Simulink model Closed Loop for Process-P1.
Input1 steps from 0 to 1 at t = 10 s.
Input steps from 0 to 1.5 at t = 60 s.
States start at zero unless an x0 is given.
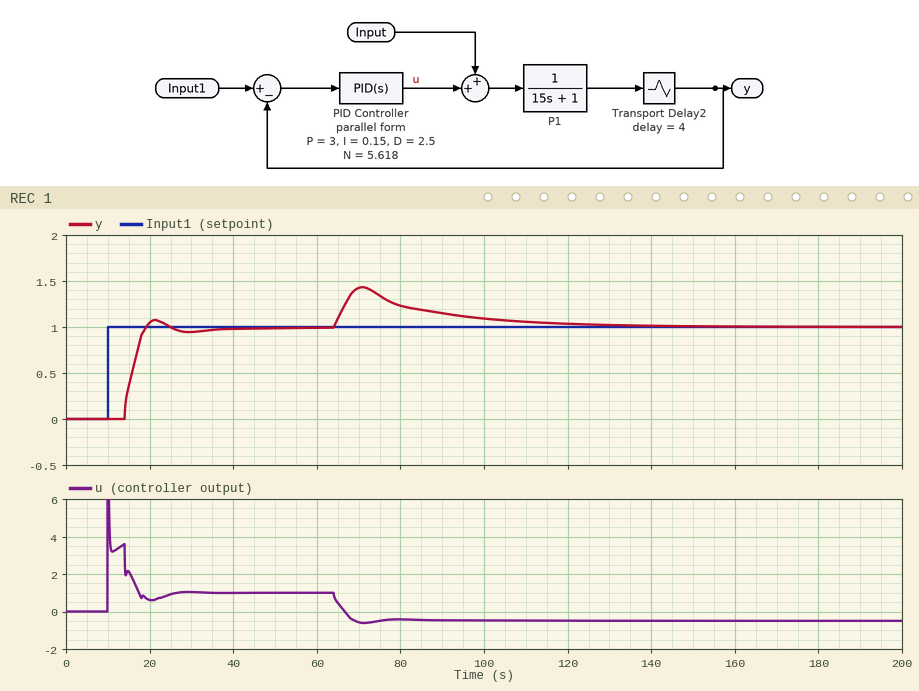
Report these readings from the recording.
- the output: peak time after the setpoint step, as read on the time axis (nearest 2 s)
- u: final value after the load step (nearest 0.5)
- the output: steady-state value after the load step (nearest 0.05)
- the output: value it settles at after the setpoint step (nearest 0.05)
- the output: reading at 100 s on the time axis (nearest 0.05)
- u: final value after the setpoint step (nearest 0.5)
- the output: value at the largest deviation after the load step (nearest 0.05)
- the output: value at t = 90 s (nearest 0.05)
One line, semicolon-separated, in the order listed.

22 s; -0.5; 1.00; 1.00; 1.10; 1.0; 1.45; 1.15
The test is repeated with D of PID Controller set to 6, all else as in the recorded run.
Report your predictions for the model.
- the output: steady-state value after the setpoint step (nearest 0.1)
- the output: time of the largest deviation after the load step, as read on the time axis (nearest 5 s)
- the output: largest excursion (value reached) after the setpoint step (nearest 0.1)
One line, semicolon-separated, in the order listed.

1.0; 70 s; 1.1
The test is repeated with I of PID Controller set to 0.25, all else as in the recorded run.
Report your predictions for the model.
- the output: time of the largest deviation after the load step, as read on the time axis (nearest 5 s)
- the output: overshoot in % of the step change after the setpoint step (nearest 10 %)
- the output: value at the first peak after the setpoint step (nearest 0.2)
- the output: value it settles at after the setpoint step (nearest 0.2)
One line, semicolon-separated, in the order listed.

70 s; 20 %; 1.2; 1.0
